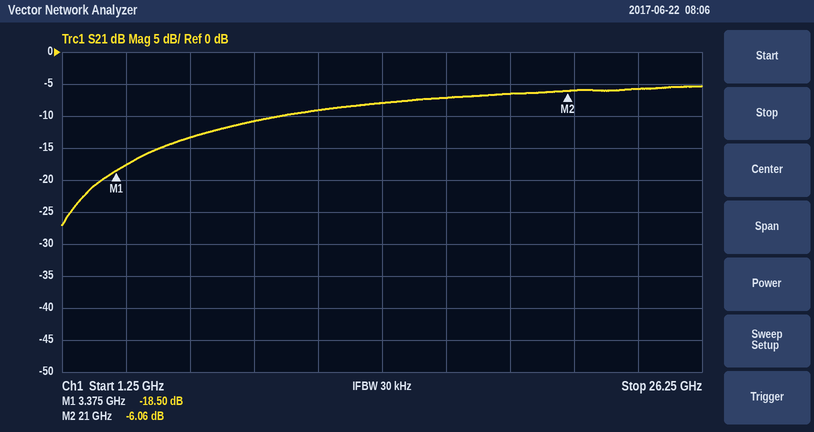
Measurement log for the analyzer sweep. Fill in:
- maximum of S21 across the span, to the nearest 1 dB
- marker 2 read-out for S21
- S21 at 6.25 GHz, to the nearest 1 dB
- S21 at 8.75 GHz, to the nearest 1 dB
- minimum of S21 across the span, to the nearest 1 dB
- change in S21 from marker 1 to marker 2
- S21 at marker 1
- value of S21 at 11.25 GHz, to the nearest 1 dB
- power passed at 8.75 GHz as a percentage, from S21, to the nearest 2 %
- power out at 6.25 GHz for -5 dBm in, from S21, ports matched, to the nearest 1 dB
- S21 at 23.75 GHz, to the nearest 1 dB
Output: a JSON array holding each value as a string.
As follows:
["-5 dB", "-6.06 dB", "-13 dB", "-11 dB", "-27 dB", "12.44 dB", "-18.50 dB", "-9 dB", "8 %", "-18 dBm", "-6 dB"]
